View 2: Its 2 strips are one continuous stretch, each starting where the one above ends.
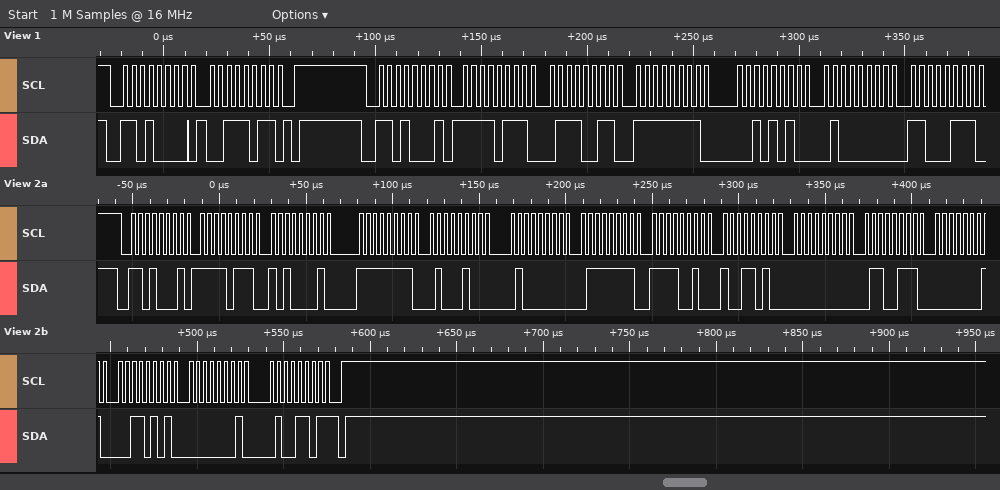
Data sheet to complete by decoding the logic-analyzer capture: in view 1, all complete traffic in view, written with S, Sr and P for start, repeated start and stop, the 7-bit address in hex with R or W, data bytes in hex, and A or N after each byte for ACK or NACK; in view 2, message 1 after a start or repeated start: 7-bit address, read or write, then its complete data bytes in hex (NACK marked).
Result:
S 68W A 3B A P S 68R A F7 A 73 A FF A 2A A 40 A C7 A
0x68 read: F7 A1 FF 44 40 7F F2 9A 00 67 01 35 01 4D NACK
